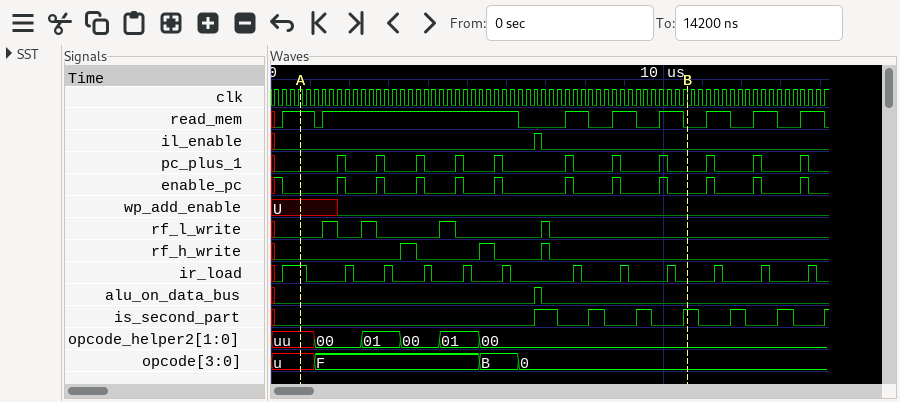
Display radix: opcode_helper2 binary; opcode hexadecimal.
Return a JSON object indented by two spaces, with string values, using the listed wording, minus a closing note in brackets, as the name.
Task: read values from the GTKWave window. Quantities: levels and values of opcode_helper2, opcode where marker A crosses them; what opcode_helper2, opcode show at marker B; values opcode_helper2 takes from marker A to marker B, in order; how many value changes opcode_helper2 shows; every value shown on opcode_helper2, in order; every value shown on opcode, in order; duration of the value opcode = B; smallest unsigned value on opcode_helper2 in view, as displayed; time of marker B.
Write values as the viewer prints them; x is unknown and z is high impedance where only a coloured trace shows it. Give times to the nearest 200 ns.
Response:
{
  "levels and values of opcode_helper2, opcode where marker A crosses them": "opcode_helper2=uu, opcode=u",
  "what opcode_helper2, opcode show at marker B": "opcode_helper2=00, opcode=0",
  "values opcode_helper2 takes from marker A to marker B, in order": "uu, 00, 01, 00, 01, 00",
  "how many value changes opcode_helper2 shows": "5",
  "every value shown on opcode_helper2, in order": "uu, 00, 01, 00, 01, 00",
  "every value shown on opcode, in order": "u, F, B, 0",
  "duration of the value opcode = B": "1000 ns",
  "smallest unsigned value on opcode_helper2 in view, as displayed": "00",
  "time of marker B": "10600 ns"
}
